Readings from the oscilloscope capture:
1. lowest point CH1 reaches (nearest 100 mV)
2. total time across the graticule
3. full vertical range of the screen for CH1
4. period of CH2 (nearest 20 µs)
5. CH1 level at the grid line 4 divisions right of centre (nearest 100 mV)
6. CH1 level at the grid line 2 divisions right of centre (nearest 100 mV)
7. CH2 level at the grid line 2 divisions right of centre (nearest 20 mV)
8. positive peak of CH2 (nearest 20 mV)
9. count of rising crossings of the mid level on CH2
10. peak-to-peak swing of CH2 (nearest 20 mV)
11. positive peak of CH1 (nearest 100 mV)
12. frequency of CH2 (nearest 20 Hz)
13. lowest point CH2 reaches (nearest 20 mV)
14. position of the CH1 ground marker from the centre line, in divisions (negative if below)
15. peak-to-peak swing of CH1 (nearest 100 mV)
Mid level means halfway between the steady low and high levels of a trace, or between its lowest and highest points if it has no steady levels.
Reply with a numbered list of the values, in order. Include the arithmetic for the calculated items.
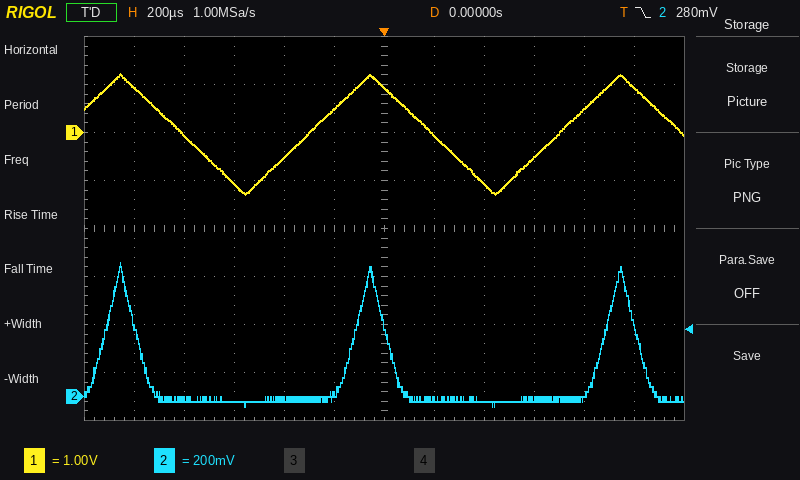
1. -1.3 V
2. 2.4 ms
3. 8 V
4. 1.00 ms
5. 500 mV
6. -1.1 V
7. -20 mV
8. 560 mV
9. 3
10. 560 mV − (-40 mV) = 600 mV
11. 1.2 V
12. 1 / 1.00 ms ≈ 1.00 kHz
13. -40 mV
14. +2.0 div
15. 1.2 V − (-1.3 V) = 2.5 V
